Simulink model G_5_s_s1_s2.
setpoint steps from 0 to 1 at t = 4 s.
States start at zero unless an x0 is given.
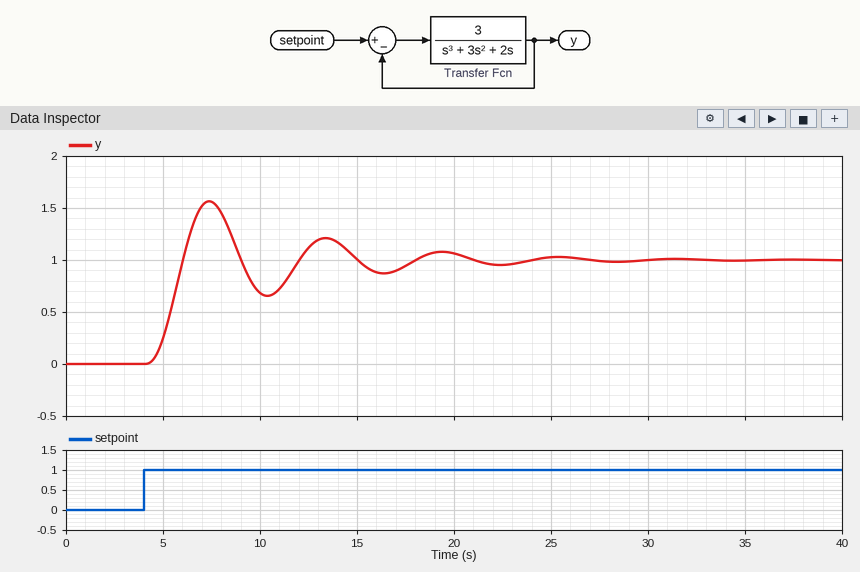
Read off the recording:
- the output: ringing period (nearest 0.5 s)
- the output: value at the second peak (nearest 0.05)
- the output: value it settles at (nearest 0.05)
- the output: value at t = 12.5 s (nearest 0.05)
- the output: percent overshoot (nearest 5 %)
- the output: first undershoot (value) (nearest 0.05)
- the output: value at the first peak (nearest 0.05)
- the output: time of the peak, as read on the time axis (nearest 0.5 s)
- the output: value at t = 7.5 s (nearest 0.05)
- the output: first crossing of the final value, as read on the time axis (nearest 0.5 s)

6.0 s
1.20
1.00
1.10
55 %
0.65
1.55
7.5 s
1.55
6.0 s
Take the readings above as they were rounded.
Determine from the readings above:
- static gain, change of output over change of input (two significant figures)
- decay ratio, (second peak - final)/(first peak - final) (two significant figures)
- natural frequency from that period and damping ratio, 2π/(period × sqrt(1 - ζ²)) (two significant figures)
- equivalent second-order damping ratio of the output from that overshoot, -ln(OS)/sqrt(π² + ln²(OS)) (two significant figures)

1.0
0.36
1.1 rad/s
0.19
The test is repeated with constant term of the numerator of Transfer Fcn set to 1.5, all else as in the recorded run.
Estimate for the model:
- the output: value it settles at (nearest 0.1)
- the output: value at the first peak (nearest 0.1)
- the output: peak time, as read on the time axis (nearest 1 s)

1.0
1.3
9 s
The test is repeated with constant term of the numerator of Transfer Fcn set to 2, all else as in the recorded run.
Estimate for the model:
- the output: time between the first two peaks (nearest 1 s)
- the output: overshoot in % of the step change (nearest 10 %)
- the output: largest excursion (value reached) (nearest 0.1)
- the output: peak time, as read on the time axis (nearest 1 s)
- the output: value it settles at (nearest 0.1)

7 s
40 %
1.4
8 s
1.0
